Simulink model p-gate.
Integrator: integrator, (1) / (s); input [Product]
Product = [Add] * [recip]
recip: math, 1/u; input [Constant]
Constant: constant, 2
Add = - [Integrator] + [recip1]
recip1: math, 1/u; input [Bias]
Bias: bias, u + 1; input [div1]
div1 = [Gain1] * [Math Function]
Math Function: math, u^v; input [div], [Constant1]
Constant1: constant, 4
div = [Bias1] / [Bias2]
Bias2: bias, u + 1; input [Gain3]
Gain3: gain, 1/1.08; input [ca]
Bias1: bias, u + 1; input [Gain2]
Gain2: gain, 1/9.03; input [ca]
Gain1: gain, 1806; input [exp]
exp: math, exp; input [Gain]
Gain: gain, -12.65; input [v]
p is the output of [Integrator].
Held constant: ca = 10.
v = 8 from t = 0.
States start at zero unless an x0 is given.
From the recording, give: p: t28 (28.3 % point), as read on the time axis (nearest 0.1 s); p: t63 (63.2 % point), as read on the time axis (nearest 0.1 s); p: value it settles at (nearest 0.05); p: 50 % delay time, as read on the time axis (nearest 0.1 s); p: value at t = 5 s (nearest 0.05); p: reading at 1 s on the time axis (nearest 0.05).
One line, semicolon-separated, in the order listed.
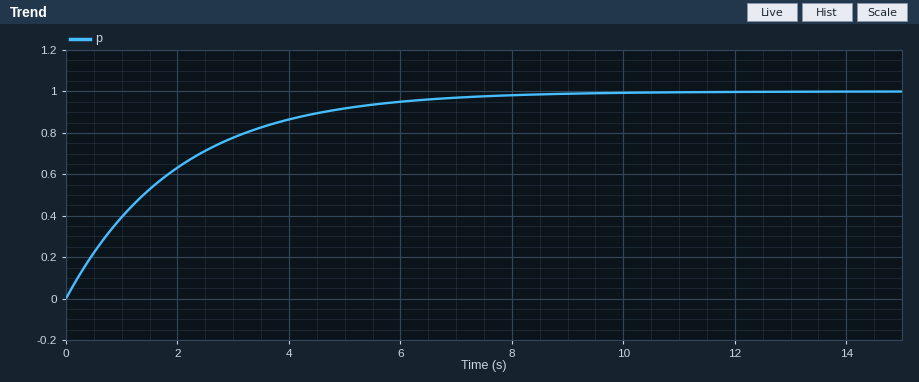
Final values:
0.7 s; 2.0 s; 1.00; 1.4 s; 0.90; 0.40
